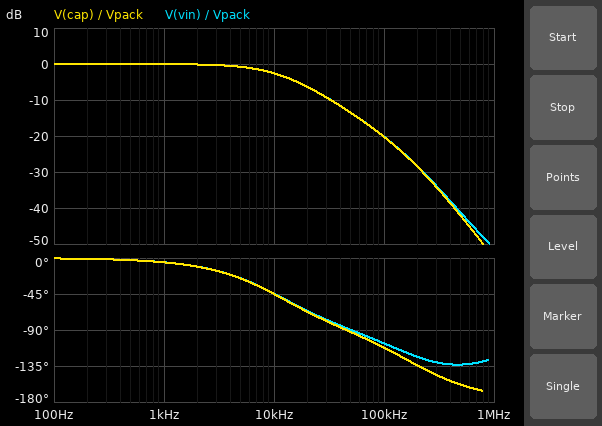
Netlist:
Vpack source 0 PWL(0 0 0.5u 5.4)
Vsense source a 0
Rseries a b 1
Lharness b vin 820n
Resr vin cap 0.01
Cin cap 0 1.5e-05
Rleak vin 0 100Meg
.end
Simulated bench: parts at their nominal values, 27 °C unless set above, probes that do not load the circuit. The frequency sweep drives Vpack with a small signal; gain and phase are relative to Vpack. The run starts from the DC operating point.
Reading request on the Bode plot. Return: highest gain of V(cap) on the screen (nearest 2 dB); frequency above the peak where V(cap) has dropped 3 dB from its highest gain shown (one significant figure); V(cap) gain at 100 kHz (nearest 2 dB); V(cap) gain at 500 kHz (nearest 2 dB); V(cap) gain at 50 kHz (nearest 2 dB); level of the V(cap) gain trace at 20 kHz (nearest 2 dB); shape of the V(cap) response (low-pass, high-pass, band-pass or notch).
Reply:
0 dB
10 kHz
-20 dB
-42 dB
-14 dB
-6 dB
low-pass
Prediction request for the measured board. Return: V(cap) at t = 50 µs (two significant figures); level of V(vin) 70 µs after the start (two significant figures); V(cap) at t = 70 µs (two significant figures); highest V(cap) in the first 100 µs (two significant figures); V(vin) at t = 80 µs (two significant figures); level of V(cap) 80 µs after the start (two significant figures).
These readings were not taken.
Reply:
5.2 V
5.4 V
5.4 V
5.4 V
5.4 V
5.4 V
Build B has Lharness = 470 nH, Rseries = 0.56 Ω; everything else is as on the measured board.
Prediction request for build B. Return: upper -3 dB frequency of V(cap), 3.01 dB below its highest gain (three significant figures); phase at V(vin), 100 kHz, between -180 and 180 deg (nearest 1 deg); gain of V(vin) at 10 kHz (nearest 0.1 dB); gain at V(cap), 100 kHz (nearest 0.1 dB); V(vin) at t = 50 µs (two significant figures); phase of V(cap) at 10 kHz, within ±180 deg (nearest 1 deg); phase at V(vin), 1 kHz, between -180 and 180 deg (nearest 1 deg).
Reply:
20.6 kHz
-103 deg
-0.9 dB
-15.1 dB
5.4 V
-29 deg
-3 deg
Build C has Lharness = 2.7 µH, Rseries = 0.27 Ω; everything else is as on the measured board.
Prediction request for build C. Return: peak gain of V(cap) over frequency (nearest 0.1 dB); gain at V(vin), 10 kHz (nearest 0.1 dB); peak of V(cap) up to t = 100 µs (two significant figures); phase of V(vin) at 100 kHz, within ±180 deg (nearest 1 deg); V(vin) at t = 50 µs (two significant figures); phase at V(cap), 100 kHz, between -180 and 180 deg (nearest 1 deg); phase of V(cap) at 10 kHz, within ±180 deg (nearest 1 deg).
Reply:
4.1 dB
1.1 dB
7.2 V
-165 deg
5.1 V
-170 deg
-17 deg
